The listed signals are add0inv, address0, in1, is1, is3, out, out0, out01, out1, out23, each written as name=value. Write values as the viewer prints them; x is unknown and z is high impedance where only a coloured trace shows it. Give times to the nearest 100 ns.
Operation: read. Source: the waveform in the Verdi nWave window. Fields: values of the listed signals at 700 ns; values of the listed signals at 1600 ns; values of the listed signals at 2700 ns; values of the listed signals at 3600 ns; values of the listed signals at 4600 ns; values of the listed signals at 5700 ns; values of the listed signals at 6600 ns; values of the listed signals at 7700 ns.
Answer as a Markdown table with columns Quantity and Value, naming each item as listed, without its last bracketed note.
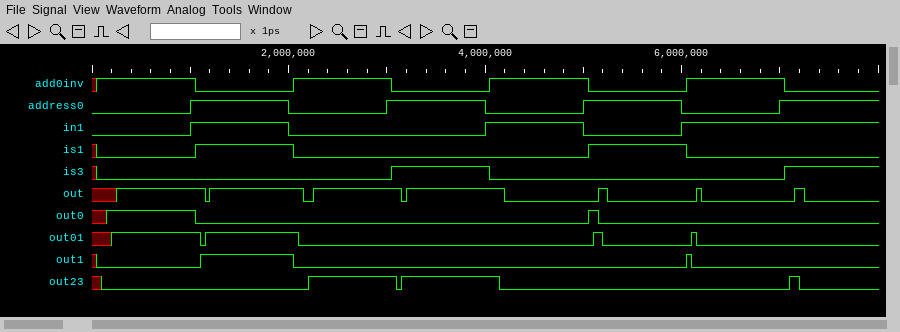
| Quantity | Value |
|---|---|
| values of the listed signals at 700 ns | add0inv=1, address0=0, in1=0, is1=0, is3=0, out=1, out0=1, out01=1, out1=0, out23=0 |
| values of the listed signals at 1600 ns | add0inv=0, address0=1, in1=1, is1=1, is3=0, out=1, out0=0, out01=1, out1=1, out23=0 |
| values of the listed signals at 2700 ns | add0inv=1, address0=0, in1=0, is1=0, is3=0, out=1, out0=0, out01=0, out1=0, out23=1 |
| values of the listed signals at 3600 ns | add0inv=0, address0=1, in1=0, is1=0, is3=1, out=1, out0=0, out01=0, out1=0, out23=1 |
| values of the listed signals at 4600 ns | add0inv=1, address0=0, in1=1, is1=0, is3=0, out=0, out0=0, out01=0, out1=0, out23=0 |
| values of the listed signals at 5700 ns | add0inv=0, address0=1, in1=0, is1=1, is3=0, out=0, out0=0, out01=0, out1=0, out23=0 |
| values of the listed signals at 6600 ns | add0inv=1, address0=0, in1=1, is1=0, is3=0, out=0, out0=0, out01=0, out1=0, out23=0 |
| values of the listed signals at 7700 ns | add0inv=0, address0=1, in1=1, is1=0, is3=1, out=0, out0=0, out01=0, out1=0, out23=0 |
